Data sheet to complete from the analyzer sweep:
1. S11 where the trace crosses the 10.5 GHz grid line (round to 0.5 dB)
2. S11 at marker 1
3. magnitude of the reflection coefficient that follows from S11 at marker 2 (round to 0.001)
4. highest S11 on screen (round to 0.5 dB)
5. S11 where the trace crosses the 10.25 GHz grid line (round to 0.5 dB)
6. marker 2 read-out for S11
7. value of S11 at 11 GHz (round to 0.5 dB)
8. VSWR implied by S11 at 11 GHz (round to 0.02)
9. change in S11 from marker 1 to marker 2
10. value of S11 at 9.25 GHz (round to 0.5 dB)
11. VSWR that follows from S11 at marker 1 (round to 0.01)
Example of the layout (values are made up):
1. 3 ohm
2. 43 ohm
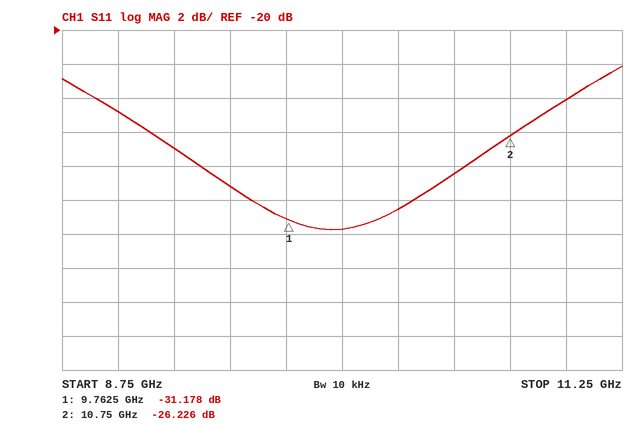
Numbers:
1. -28.5 dB
2. -31.178 dB
3. 0.049
4. -22.0 dB
5. -30.5 dB
6. -26.226 dB
7. -24.0 dB
8. 1.14
9. 4.952 dB
10. -27.0 dB
11. 1.06
